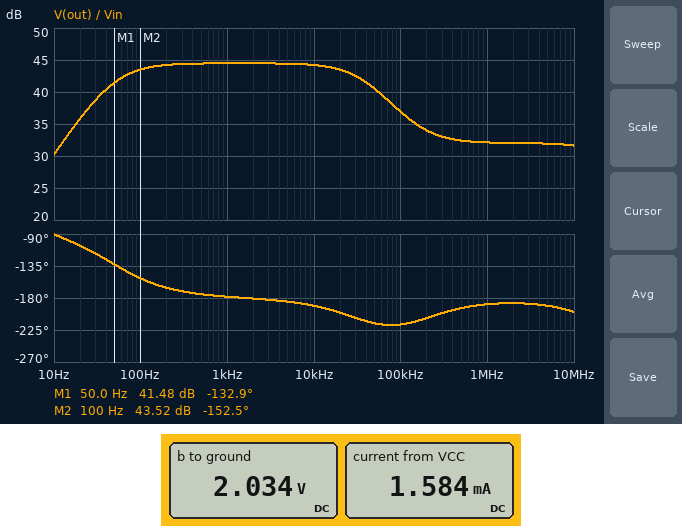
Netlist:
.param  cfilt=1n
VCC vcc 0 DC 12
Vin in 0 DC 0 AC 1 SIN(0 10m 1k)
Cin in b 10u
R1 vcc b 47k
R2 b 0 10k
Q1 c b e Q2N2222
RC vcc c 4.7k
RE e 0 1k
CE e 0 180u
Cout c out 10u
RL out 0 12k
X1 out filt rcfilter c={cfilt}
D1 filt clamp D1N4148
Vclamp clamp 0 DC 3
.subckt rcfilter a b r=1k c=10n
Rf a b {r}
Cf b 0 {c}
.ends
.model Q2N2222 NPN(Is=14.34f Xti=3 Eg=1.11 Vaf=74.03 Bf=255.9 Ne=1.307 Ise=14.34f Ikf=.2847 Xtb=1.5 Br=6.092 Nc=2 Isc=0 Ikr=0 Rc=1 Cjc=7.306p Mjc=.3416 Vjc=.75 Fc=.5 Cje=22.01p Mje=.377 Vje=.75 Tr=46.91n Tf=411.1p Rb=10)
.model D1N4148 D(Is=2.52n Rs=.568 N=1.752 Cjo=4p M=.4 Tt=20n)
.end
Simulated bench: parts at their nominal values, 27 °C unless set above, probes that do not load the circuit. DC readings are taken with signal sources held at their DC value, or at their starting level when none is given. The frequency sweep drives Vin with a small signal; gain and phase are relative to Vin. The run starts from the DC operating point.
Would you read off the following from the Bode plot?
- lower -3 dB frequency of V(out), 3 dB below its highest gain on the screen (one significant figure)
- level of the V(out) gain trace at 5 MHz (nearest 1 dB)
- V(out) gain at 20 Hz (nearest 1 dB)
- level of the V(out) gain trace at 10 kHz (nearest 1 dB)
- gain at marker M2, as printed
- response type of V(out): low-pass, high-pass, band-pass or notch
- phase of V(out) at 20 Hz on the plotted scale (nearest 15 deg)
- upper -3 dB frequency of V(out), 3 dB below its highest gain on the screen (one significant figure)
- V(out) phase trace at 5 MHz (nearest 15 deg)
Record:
50 Hz
32 dB
36 dB
44 dB
43.52 dB
band-pass
-105 deg
40 kHz
-195 deg
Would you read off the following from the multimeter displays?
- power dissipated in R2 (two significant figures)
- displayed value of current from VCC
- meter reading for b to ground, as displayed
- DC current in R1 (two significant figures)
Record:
410 µW
1.584 mA
2.034 V
210 µA
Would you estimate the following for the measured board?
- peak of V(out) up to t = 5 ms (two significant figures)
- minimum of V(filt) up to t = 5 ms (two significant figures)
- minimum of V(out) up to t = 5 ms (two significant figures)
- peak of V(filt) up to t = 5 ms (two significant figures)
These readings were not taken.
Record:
1.5 V
-1.9 V
-1.9 V
1.5 V
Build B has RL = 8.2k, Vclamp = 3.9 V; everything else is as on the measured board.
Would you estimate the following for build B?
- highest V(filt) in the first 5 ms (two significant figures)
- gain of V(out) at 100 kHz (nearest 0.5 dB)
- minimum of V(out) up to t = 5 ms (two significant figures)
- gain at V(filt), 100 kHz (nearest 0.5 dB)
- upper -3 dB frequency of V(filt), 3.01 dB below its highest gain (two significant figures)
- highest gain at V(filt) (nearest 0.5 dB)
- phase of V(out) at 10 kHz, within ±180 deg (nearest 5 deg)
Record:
1.3 V
36.5 dB
-1.7 V
35.0 dB
41 kHz
43.5 dB
170 deg
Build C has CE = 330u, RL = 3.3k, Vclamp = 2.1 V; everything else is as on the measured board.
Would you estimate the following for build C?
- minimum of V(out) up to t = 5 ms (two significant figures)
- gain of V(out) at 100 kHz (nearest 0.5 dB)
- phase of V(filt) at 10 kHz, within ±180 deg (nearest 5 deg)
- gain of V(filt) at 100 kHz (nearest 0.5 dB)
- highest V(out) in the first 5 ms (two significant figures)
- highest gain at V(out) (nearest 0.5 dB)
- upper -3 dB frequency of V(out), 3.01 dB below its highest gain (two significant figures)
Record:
-1.1 V
35.0 dB
170 deg
33.5 dB
880 mV
40.0 dB
63 kHz
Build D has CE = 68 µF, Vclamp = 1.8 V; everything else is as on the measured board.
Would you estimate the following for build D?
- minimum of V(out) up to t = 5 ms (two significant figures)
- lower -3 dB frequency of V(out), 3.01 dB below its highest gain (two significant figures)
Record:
-1.8 V
120 Hz
